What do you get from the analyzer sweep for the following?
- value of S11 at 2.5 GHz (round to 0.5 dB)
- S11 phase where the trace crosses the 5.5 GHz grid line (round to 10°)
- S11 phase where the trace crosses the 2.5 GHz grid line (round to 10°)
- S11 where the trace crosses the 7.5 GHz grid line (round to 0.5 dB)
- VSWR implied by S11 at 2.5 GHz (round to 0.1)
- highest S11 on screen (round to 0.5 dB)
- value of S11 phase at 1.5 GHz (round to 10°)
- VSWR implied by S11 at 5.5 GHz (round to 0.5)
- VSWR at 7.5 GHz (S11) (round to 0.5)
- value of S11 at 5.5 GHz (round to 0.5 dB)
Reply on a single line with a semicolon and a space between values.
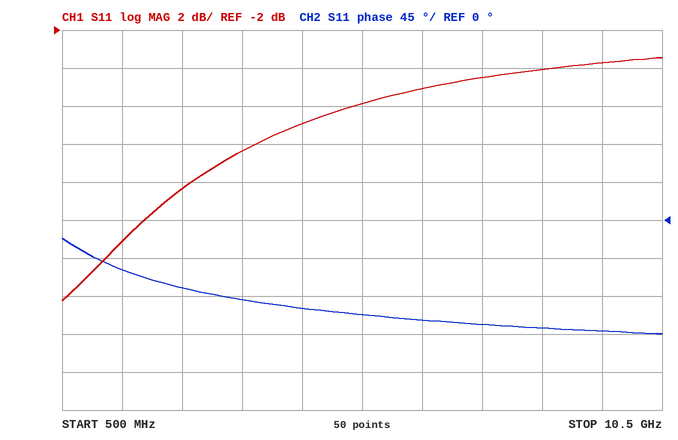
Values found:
-10.5 dB; -110°; -80°; -4.5 dB; 1.9; -3.5 dB; -60°; 3.0; 4.0; -6.0 dB
